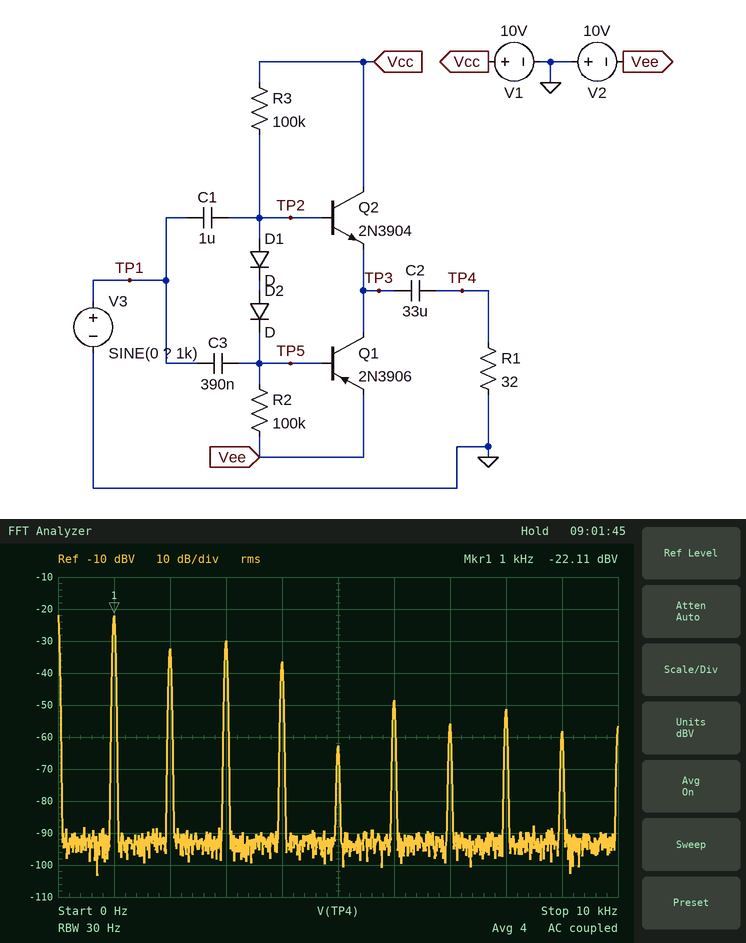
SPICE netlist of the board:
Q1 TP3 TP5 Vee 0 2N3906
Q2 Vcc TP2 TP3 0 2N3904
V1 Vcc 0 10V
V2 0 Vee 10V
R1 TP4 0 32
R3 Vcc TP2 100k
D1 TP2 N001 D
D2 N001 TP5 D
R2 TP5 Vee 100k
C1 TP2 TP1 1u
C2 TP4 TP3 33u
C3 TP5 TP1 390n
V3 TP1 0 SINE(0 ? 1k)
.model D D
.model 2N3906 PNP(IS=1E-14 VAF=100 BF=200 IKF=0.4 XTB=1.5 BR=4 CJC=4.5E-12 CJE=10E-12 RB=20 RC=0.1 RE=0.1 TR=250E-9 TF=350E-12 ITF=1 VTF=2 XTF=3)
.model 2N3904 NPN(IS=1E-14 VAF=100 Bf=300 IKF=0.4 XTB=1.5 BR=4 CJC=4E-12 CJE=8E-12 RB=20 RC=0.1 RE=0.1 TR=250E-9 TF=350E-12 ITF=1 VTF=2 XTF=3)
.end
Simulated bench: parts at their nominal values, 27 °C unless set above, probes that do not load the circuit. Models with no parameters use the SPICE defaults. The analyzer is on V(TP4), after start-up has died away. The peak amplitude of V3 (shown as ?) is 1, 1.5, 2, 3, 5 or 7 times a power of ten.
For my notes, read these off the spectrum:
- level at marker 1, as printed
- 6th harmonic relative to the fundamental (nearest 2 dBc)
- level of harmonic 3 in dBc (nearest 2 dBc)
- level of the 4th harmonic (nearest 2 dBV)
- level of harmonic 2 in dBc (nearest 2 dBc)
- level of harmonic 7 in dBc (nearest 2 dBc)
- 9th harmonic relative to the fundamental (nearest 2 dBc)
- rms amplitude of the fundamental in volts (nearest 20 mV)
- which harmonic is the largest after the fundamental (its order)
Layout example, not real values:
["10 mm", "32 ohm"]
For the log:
["-22.11 dBV", "-26 dBc", "-8 dBc", "-36 dBV", "-10 dBc", "-34 dBc", "-36 dBc", "80 mV", "3"]
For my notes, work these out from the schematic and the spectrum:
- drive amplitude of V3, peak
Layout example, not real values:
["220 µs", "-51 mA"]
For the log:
["700 mV"]
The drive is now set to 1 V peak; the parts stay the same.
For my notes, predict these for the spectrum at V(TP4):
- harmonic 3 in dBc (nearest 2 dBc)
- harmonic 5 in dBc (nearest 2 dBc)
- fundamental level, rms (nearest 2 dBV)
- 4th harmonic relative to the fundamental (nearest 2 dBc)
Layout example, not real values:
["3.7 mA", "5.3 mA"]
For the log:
["-6 dBc", "-22 dBc", "-22 dBV", "-12 dBc"]
